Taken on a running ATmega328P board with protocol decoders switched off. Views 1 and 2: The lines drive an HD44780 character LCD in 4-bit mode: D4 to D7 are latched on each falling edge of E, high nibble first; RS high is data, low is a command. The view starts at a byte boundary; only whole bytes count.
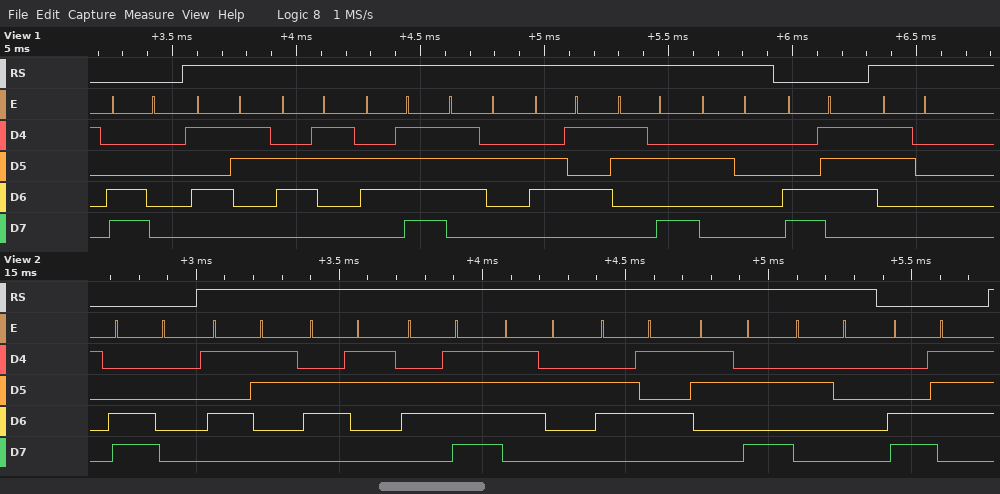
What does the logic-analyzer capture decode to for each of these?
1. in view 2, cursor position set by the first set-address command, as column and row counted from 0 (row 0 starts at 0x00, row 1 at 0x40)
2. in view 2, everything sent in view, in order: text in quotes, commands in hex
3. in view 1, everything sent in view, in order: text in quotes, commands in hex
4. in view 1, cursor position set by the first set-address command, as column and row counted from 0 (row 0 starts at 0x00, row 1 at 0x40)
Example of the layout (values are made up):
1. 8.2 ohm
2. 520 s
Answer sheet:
1. column 0, row 1
2. 0xC0 "Score: " 0xC7
3. 0xC0 "Score: " 0xC7 "0"
4. column 0, row 1
